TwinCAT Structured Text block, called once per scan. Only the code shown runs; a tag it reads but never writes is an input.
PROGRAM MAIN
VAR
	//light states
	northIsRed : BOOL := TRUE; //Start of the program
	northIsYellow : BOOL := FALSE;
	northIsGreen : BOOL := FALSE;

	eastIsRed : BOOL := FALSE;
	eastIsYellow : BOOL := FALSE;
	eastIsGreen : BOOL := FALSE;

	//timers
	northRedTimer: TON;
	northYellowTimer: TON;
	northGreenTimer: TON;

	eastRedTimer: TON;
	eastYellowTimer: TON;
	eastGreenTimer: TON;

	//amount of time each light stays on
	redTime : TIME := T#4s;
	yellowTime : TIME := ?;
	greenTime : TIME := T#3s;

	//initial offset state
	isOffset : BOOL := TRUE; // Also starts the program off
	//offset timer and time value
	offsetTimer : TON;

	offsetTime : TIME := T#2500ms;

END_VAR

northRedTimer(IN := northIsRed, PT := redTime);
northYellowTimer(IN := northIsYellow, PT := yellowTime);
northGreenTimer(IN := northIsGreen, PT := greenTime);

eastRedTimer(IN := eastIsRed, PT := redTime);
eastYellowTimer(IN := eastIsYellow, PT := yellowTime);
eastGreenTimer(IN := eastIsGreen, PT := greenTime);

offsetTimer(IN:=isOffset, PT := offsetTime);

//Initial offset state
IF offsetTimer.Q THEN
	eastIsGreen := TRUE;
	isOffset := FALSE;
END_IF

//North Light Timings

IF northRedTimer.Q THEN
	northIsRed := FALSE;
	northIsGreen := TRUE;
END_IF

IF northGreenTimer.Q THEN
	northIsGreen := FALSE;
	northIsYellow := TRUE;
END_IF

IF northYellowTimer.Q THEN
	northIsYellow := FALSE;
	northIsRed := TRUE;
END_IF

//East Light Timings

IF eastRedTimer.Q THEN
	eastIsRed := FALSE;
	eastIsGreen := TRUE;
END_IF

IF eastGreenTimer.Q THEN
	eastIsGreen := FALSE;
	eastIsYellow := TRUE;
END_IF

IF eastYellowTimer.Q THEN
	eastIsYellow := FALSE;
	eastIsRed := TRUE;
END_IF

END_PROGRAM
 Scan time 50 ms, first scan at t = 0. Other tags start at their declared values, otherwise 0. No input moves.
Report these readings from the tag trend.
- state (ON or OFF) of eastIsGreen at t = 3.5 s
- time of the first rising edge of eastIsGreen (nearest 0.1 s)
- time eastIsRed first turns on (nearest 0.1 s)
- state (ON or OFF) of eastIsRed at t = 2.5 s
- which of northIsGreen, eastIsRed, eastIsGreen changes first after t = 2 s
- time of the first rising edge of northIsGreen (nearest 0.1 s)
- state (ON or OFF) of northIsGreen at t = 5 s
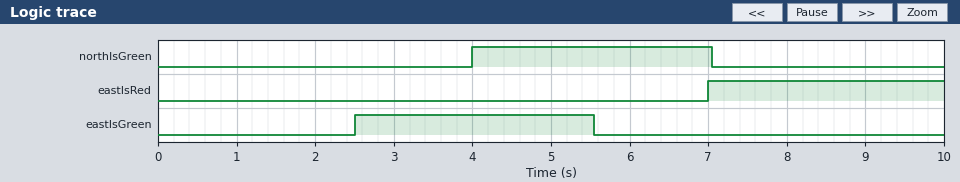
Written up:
ON
2.5 s
7.0 s
OFF
eastIsGreen
4.0 s
ON
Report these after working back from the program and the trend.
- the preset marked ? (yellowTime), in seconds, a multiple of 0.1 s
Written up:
1.4 s
